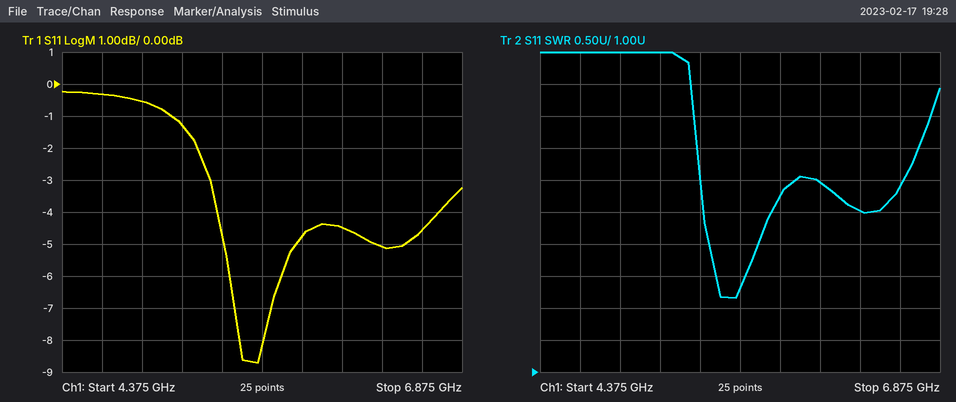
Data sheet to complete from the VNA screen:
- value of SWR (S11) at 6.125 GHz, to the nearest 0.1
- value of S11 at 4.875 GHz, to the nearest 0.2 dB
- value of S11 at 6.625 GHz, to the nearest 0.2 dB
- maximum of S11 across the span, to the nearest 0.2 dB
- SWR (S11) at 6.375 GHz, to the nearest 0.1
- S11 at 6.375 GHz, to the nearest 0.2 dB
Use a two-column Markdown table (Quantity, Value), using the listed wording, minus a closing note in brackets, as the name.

| Quantity | Value |
|---|---|
| value of SWR (S11) at 6.125 GHz, to the nearest 0.1 | 4.0 |
| value of S11 at 4.875 GHz, to the nearest 0.2 dB | -0.6 dB |
| value of S11 at 6.625 GHz, to the nearest 0.2 dB | -4.6 dB |
| maximum of S11 across the span, to the nearest 0.2 dB | -0.2 dB |
| SWR (S11) at 6.375 GHz, to the nearest 0.1 | 3.5 |
| S11 at 6.375 GHz, to the nearest 0.2 dB | -5.0 dB |
